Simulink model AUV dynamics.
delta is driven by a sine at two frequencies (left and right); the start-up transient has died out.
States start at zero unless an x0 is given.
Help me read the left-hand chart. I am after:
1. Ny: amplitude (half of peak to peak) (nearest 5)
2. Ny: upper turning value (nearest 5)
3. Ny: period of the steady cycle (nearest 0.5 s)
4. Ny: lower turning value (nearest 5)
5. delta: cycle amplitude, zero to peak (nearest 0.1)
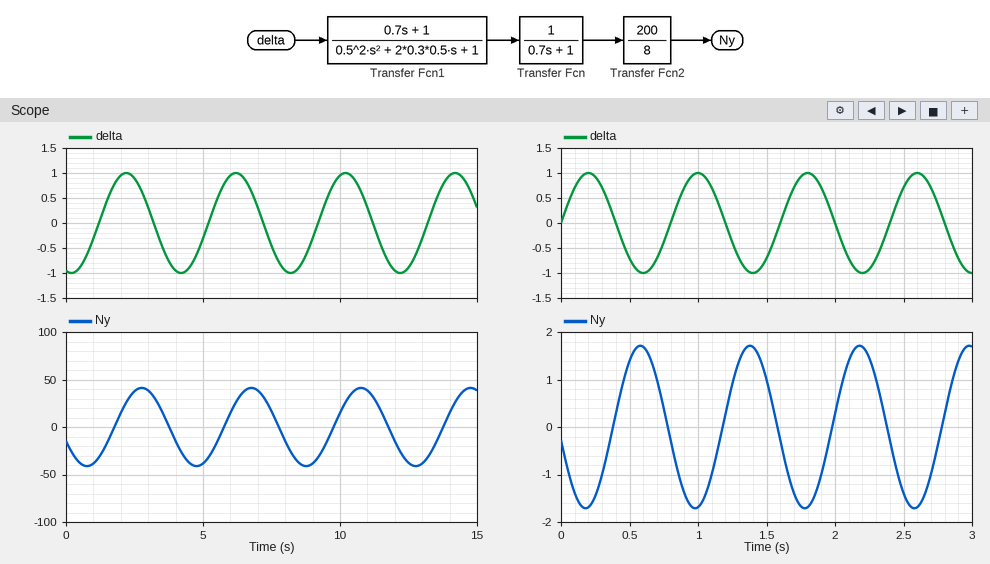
40
40
4.0 s
-40
1.0
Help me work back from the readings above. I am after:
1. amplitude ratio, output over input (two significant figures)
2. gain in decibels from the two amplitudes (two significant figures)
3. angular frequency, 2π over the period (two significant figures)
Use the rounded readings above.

40
32 dB
1.6 rad/s
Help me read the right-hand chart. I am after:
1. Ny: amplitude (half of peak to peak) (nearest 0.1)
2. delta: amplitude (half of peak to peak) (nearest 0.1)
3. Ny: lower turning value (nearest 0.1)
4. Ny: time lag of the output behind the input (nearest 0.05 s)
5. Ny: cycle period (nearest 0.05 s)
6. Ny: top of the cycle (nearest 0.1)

1.7
1.0
-1.7
0.40 s
0.80 s
1.7
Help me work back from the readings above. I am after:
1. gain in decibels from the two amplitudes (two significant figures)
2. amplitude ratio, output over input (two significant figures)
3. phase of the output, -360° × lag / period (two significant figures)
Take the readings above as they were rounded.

4.6 dB
1.7
-180°
